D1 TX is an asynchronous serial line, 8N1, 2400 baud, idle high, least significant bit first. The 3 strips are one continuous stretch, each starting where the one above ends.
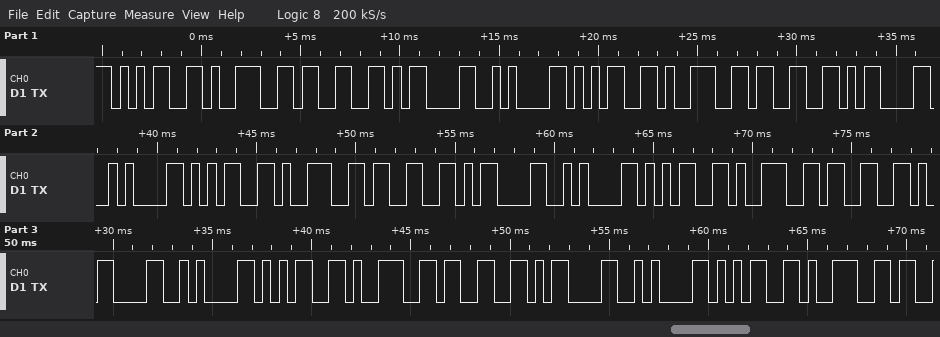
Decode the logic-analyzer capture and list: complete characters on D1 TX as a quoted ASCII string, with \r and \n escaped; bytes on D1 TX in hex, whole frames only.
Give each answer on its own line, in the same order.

"593\r\n593\r\n593\r\n593\r\n593\r\n59"
35 39 33 0D 0A 35 39 33 0D 0A 35 39 33 0D 0A 35 39 33 0D 0A 35 39 33 0D 0A 35 39
